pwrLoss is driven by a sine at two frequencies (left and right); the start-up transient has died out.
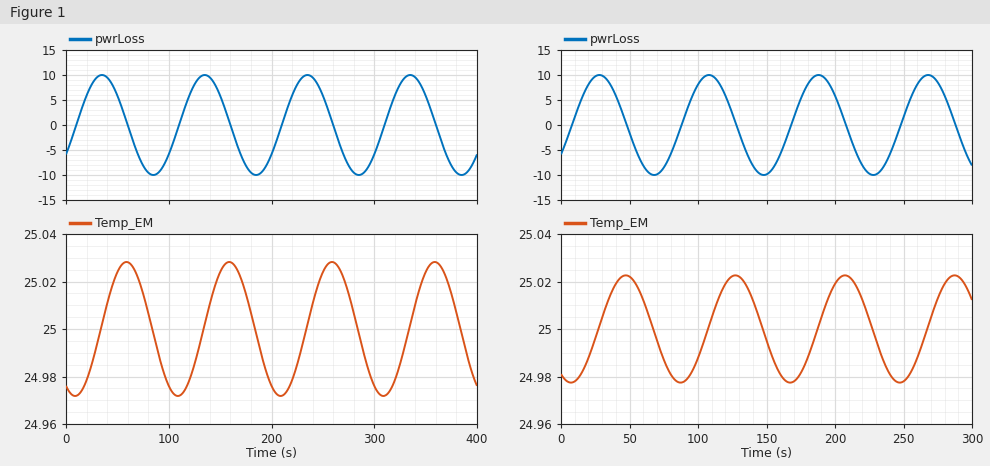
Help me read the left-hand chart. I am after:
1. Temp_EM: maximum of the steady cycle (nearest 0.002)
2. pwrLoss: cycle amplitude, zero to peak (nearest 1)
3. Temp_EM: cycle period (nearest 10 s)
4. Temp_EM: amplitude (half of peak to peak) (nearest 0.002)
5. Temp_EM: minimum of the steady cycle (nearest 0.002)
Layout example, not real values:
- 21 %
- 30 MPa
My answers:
- 25.028
- 10
- 100 s
- 0.028
- 24.972
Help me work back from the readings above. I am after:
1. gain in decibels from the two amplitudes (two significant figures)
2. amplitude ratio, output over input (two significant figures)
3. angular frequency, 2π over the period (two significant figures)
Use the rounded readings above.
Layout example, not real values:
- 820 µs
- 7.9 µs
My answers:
- -51 dB
- 0.0028
- 0.063 rad/s
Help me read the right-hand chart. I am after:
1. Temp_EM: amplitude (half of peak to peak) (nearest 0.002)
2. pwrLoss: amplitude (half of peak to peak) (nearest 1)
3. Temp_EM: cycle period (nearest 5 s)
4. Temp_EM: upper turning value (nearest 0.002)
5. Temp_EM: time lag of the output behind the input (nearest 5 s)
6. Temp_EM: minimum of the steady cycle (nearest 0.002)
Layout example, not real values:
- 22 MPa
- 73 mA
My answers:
- 0.022
- 10
- 80 s
- 25.022
- 20 s
- 24.978
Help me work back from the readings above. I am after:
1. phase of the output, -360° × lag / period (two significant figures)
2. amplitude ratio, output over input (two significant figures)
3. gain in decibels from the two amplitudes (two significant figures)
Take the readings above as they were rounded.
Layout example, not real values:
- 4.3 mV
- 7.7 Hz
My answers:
- -90°
- 0.0022
- -53 dB
